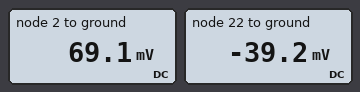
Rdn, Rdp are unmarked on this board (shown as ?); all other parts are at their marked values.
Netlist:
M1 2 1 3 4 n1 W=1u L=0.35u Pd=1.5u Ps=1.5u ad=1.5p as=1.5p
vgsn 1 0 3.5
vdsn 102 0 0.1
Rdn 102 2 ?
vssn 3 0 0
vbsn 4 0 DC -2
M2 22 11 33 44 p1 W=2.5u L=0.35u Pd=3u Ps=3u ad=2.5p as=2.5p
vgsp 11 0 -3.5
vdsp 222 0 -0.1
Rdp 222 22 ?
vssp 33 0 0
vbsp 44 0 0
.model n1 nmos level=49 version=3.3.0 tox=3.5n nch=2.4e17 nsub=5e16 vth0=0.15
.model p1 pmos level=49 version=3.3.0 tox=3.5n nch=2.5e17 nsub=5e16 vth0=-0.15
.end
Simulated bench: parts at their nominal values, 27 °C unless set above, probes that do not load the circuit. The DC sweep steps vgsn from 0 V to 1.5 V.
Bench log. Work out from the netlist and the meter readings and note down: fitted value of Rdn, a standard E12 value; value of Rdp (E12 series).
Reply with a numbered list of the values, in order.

1. 390 Ω
2. 1.2 kΩ
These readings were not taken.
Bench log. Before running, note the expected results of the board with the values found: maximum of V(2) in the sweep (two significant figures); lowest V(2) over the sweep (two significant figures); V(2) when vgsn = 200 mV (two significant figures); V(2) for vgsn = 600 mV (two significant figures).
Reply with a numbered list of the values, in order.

1. 100 mV
2. 82 mV
3. 100 mV
4. 100 mV
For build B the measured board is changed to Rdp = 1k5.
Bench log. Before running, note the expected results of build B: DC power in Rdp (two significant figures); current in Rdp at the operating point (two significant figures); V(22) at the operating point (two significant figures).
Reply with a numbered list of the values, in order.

1. 2.9 µW
2. 44 µA
3. -34 mV
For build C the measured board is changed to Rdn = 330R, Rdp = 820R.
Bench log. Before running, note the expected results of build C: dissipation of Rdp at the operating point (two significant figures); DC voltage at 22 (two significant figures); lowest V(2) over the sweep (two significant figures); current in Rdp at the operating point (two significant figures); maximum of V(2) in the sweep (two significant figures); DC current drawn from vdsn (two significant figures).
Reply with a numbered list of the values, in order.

1. 3.2 µW
2. -49 mV
3. 84 mV
4. 63 µA
5. 100 mV
6. 83 µA
